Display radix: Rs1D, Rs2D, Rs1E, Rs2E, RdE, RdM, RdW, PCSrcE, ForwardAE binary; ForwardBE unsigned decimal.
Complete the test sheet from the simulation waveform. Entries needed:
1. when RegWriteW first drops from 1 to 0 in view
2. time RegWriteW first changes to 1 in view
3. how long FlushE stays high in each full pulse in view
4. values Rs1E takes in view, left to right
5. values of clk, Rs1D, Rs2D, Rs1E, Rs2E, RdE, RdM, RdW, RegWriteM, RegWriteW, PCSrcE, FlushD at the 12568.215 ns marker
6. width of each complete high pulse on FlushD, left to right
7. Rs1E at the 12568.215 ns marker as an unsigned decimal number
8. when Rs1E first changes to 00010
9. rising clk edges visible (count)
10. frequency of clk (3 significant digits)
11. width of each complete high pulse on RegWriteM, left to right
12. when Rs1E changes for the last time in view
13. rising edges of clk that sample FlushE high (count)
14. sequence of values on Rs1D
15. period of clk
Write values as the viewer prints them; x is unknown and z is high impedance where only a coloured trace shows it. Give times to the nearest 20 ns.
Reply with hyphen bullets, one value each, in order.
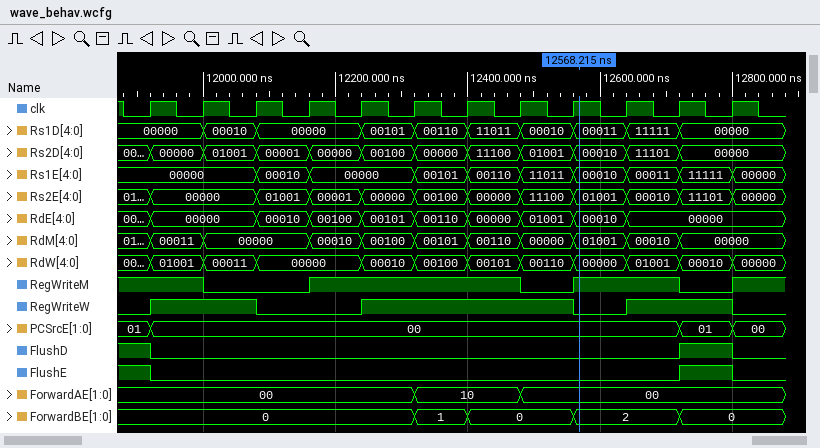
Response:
- 12080 ns
- 11920 ns
- 80 ns
- 00000, 00010, 00000, 00101, 00110, 11011, 00010, 00011, 11111, 00000
- clk=1, Rs1D=00011, Rs2D=00010, Rs1E=00010, Rs2E=01001, RdE=00010, RdM=01001, RdW=00000, RegWriteM=1, RegWriteW=0, PCSrcE=00, FlushD=0
- 80 ns
- 2
- 12080 ns
- 12
- 12.5 MHz
- 320 ns, 160 ns
- 12800 ns
- 2
- 00000, 00010, 00000, 00101, 00110, 11011, 00010, 00011, 11111, 00000
- 80 ns
